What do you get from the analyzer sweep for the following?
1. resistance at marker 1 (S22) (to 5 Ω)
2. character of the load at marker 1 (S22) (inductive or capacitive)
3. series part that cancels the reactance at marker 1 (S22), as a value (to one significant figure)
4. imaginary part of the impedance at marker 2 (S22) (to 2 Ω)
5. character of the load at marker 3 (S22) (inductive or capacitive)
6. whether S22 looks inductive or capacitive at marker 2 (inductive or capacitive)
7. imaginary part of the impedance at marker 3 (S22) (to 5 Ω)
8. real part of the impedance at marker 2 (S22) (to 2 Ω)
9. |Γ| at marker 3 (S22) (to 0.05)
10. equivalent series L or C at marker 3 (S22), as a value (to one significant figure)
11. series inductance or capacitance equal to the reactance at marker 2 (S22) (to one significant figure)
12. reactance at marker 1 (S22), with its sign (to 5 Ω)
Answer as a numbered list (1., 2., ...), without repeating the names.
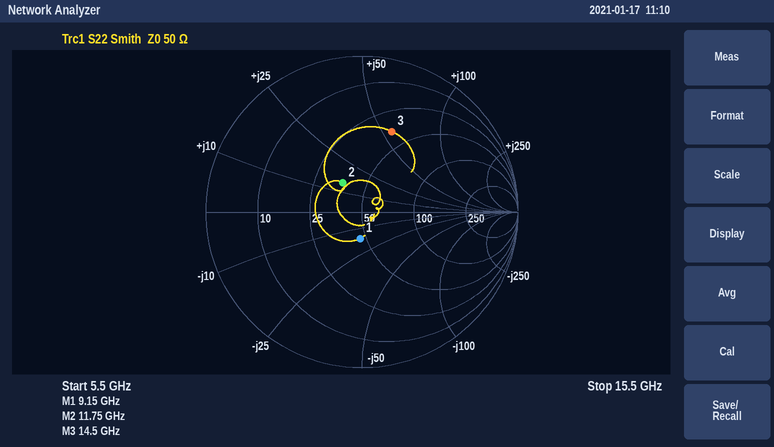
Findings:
1. 45 Ω
2. capacitive
3. 300 pH
4. +14 Ω
5. inductive
6. inductive
7. +55 Ω
8. 36 Ω
9. 0.55
10. 600 pH
11. 200 pH
12. -15 Ω
